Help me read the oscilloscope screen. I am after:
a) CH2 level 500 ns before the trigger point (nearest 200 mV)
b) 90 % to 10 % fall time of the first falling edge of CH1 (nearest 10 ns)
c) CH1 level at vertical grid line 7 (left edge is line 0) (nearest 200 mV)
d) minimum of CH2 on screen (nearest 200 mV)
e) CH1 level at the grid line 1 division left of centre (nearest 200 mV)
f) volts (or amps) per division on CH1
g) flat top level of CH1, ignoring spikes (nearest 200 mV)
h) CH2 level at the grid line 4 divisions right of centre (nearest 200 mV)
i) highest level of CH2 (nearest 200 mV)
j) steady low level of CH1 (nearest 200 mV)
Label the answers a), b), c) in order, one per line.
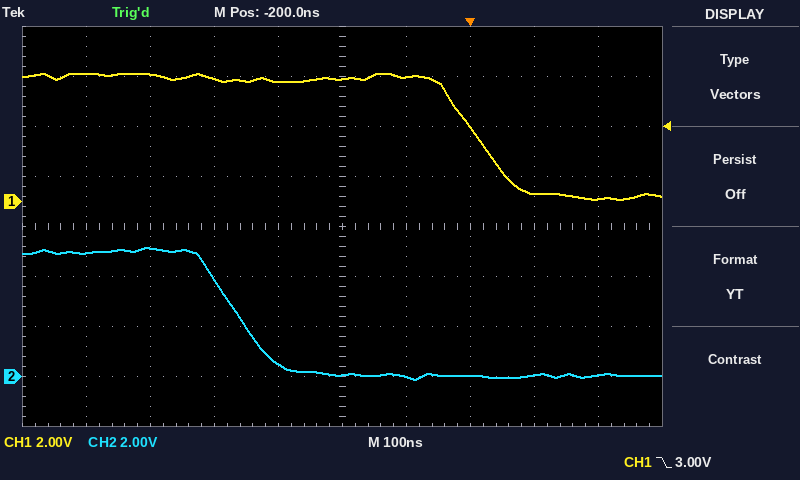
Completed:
a) 5.2 V
b) 110 ns
c) 3.0 V
d) -200 mV
e) 4.8 V
f) 2 V
g) 5.0 V
h) 0.0 V
i) 5.2 V
j) 200 mV
